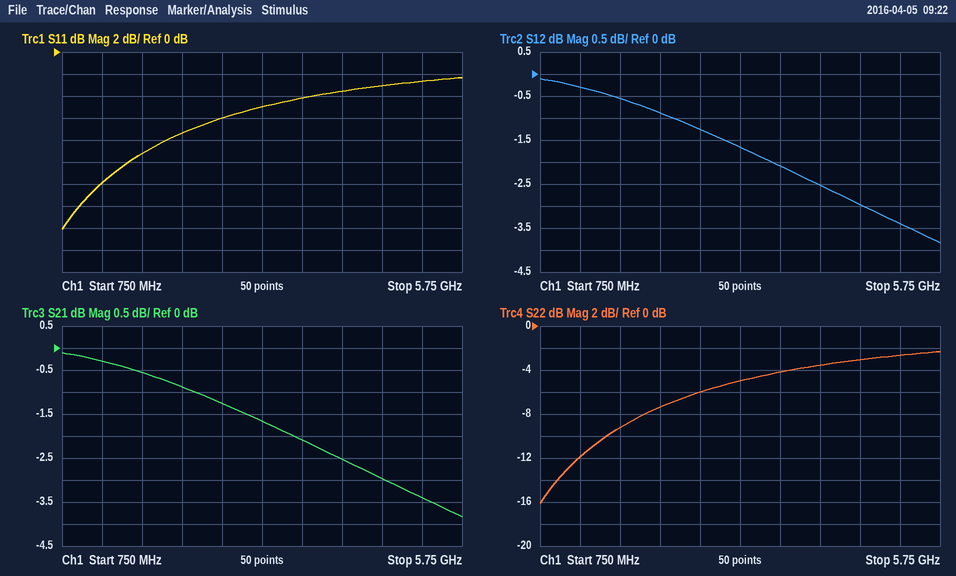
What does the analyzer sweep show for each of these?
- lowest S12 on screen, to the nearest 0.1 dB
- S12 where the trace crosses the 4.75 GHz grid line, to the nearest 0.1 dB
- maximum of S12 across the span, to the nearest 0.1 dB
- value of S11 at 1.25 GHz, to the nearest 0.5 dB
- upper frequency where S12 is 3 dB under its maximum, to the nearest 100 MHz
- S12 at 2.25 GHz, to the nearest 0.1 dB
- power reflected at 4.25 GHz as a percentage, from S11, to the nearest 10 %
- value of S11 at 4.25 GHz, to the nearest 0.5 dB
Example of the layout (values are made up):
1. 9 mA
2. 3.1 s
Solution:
1. -3.8 dB
2. -3.0 dB
3. -0.1 dB
4. -12.0 dB
5. 4.9 GHz
6. -0.9 dB
7. 40 %
8. -3.5 dB
